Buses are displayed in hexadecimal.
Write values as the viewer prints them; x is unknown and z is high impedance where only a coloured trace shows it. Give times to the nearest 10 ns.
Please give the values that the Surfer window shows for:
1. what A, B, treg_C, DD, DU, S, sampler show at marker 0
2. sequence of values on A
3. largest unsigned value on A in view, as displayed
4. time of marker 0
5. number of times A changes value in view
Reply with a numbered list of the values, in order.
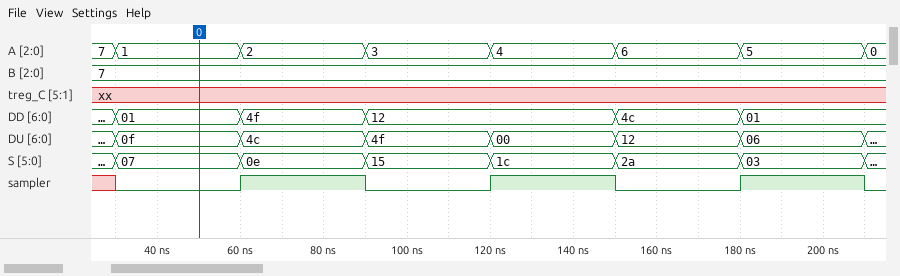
1. A=1, B=7, treg_C=xx, DD=01, DU=0f, S=07, sampler=0
2. 7, 1, 2, 3, 4, 6, 5, 0
3. 7
4. 50 ns
5. 7
